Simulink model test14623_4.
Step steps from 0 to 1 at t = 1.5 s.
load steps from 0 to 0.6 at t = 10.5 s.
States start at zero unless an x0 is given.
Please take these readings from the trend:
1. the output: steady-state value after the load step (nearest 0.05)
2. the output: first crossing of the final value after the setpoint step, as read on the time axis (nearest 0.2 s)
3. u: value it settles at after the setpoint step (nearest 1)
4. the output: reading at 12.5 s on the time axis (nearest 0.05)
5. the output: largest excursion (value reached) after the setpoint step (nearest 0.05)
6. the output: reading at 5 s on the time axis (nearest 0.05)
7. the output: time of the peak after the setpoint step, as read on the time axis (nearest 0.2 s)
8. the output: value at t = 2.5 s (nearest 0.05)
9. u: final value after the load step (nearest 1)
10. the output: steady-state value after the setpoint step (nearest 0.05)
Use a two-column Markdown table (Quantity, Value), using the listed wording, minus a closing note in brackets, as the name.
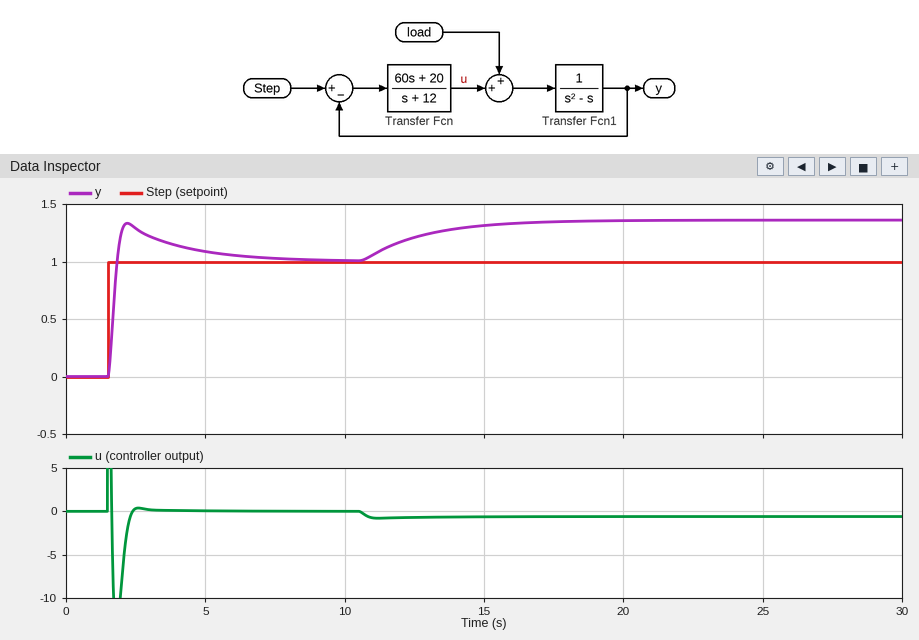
| Quantity | Value |
|---|---|
| the output: steady-state value after the load step | 1.35 |
| the output: first crossing of the final value after the setpoint step, as read on the time axis | 1.8 s |
| u: value it settles at after the setpoint step | 0 |
| the output: reading at 12.5 s on the time axis | 1.20 |
| the output: largest excursion (value reached) after the setpoint step | 1.35 |
| the output: reading at 5 s on the time axis | 1.10 |
| the output: time of the peak after the setpoint step, as read on the time axis | 2.2 s |
| the output: value at t = 2.5 s | 1.30 |
| u: final value after the load step | -1 |
| the output: steady-state value after the setpoint step | 1.00 |
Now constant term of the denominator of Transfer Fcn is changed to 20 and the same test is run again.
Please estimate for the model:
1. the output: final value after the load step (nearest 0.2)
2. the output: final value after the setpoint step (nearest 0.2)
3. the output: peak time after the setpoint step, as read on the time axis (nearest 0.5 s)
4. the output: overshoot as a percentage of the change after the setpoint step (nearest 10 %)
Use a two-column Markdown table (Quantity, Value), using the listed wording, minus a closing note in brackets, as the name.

| Quantity | Value |
|---|---|
| the output: final value after the load step | 1.6 |
| the output: final value after the setpoint step | 1.0 |
| the output: peak time after the setpoint step, as read on the time axis | 3.0 s |
| the output: overshoot as a percentage of the change after the setpoint step | 50 % |
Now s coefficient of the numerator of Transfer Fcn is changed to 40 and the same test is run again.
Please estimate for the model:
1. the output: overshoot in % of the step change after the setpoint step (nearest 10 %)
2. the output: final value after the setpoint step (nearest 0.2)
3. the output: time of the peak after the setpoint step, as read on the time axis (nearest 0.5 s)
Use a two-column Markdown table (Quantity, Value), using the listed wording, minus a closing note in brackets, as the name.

| Quantity | Value |
|---|---|
| the output: overshoot in % of the step change after the setpoint step | 50 % |
| the output: final value after the setpoint step | 1.0 |
| the output: time of the peak after the setpoint step, as read on the time axis | 2.5 s |
